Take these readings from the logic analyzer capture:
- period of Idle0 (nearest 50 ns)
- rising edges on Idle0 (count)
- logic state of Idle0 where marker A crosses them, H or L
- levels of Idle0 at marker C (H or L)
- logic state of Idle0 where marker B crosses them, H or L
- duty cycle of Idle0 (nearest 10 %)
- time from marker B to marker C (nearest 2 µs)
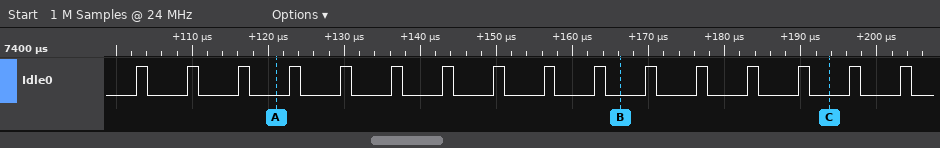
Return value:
6700 ns
16
Idle0=L
Idle0=L
Idle0=L
20 %
28 µs
